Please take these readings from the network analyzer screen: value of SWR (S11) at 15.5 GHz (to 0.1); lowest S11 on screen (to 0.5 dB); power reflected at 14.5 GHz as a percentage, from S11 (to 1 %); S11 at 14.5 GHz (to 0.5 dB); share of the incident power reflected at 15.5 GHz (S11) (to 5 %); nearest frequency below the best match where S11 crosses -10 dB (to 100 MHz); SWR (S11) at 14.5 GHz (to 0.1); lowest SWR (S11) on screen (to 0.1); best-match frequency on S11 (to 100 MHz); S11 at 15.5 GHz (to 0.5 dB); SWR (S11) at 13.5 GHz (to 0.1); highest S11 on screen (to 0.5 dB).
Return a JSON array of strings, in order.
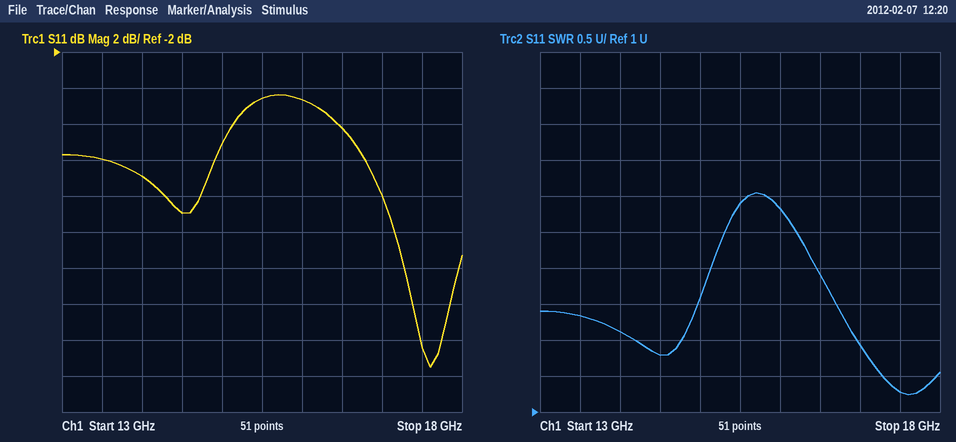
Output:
["3.9", "-19.5 dB", "8 %", "-11.0 dB", "35 %", "17.0 GHz", "1.8", "1.2", "17.6 GHz", "-4.5 dB", "2.3", "-4.5 dB"]
